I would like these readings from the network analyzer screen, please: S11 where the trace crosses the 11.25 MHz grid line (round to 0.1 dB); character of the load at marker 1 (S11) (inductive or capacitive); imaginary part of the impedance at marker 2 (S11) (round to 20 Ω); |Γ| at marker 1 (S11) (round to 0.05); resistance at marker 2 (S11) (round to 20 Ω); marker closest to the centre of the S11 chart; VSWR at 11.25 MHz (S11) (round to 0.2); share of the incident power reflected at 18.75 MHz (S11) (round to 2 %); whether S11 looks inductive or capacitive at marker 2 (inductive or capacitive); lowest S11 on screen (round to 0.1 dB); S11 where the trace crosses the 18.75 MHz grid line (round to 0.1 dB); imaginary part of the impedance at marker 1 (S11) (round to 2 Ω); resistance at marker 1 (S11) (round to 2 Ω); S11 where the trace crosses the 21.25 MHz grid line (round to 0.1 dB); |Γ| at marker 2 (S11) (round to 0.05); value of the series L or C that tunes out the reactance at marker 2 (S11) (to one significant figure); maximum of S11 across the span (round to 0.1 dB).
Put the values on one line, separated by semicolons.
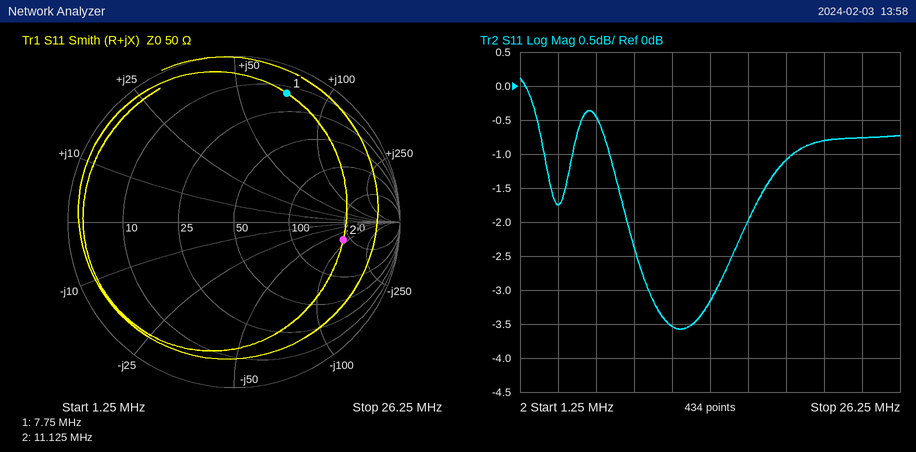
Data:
-3.5 dB; inductive; -80 Ω; 0.85; 220 Ω; marker 2; 5.0; 78 %; capacitive; -3.6 dB; -1.1 dB; +72 Ω; 14 Ω; -0.8 dB; 0.65; 1 µH; 0.1 dB
